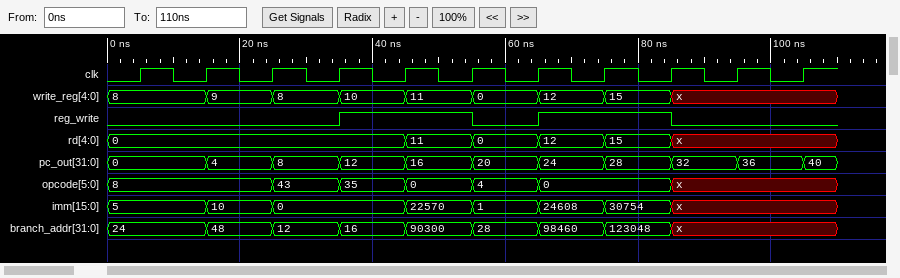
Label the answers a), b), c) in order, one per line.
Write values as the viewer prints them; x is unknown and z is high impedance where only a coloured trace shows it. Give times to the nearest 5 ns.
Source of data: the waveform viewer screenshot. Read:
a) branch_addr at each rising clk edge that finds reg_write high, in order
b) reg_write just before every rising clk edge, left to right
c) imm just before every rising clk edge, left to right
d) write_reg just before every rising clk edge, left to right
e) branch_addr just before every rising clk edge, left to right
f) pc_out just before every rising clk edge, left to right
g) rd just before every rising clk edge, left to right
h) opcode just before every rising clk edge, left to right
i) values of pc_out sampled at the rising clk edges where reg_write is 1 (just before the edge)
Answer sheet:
a) 16, 90300, 98460, 123048
b) 0 0 0 0 1 1 0 1 1 0 0
c) 5, 5, 10, 0, 0, 22570, 1, 24608, 30754, x, x
d) 8, 8, 9, 8, 10, 11, 0, 12, 15, x, x
e) 24, 24, 48, 12, 16, 90300, 28, 98460, 123048, x, x
f) 0, 0, 4, 8, 12, 16, 20, 24, 28, 32, 36
g) 0, 0, 0, 0, 0, 11, 0, 12, 15, x, x
h) 8, 8, 8, 43, 35, 0, 4, 0, 0, x, x
i) 12, 16, 24, 28
